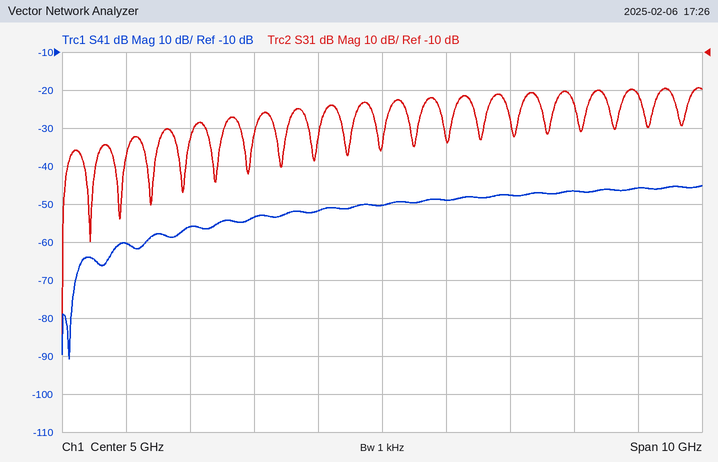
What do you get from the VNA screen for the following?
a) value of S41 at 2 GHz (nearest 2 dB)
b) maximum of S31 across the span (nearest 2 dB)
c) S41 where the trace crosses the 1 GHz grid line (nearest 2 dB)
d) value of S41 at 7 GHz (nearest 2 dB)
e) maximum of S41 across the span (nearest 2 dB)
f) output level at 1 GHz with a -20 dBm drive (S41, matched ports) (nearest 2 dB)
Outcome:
-56 dB
-20 dB
-60 dB
-48 dB
-46 dB
-80 dBm
